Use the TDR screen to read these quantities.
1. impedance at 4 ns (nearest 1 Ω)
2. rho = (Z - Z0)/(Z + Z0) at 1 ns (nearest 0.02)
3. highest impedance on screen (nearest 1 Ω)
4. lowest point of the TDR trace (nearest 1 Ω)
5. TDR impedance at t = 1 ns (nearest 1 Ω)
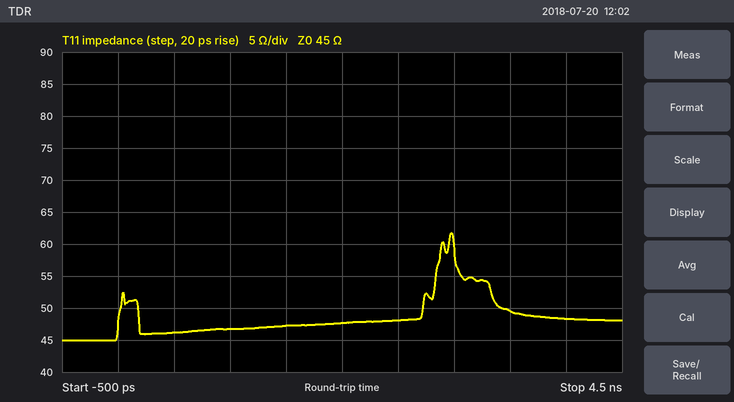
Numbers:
48 Ω
+0.02
62 Ω
45 Ω
47 Ω
